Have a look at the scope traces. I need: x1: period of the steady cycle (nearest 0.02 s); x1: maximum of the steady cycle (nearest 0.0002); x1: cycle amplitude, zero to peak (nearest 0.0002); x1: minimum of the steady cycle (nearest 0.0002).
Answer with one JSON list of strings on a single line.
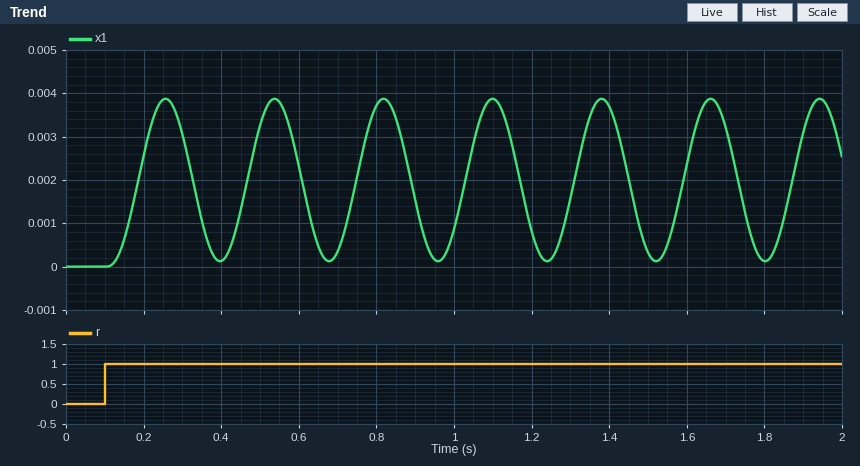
["0.28 s", "0.0038", "0.0018", "0.0002"]
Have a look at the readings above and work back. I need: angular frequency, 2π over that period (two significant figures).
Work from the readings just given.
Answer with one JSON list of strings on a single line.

["22 rad/s"]
